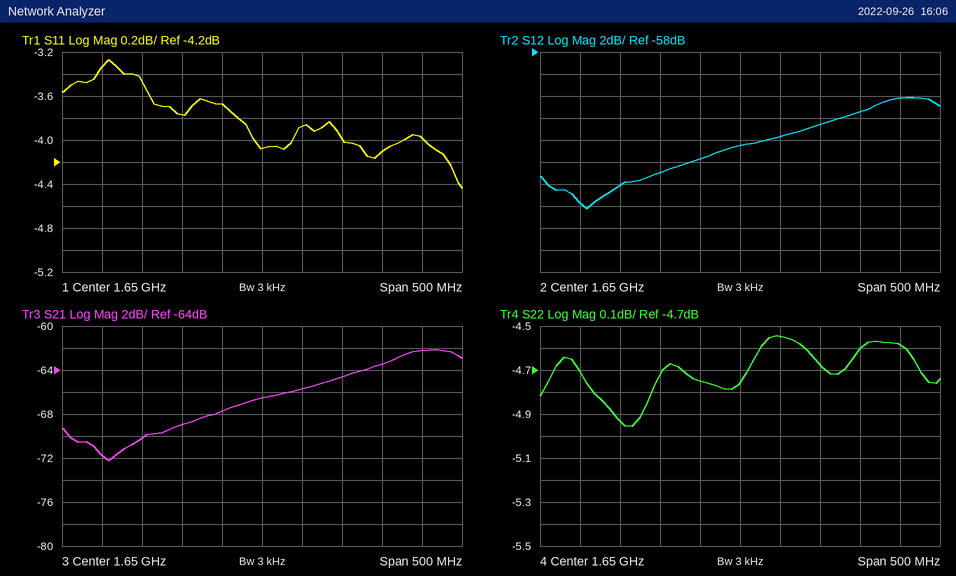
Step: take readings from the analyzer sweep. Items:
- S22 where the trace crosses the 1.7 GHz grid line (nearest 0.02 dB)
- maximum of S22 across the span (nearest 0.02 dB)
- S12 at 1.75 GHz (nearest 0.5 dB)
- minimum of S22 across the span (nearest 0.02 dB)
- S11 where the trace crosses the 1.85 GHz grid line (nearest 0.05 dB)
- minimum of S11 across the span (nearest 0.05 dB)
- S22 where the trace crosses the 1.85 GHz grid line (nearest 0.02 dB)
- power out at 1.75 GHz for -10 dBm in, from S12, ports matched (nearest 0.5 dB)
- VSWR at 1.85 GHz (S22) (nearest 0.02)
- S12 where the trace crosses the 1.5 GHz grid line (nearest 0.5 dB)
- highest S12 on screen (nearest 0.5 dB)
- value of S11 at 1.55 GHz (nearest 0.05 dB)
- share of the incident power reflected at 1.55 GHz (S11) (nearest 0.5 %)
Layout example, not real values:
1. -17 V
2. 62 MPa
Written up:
1. -4.54 dB
2. -4.54 dB
3. -64.5 dB
4. -4.96 dB
5. -4.00 dB
6. -4.45 dB
7. -4.58 dB
8. -74.5 dBm
9. 3.88
10. -70.0 dB
11. -62.0 dB
12. -3.75 dB
13. 42.0 %
